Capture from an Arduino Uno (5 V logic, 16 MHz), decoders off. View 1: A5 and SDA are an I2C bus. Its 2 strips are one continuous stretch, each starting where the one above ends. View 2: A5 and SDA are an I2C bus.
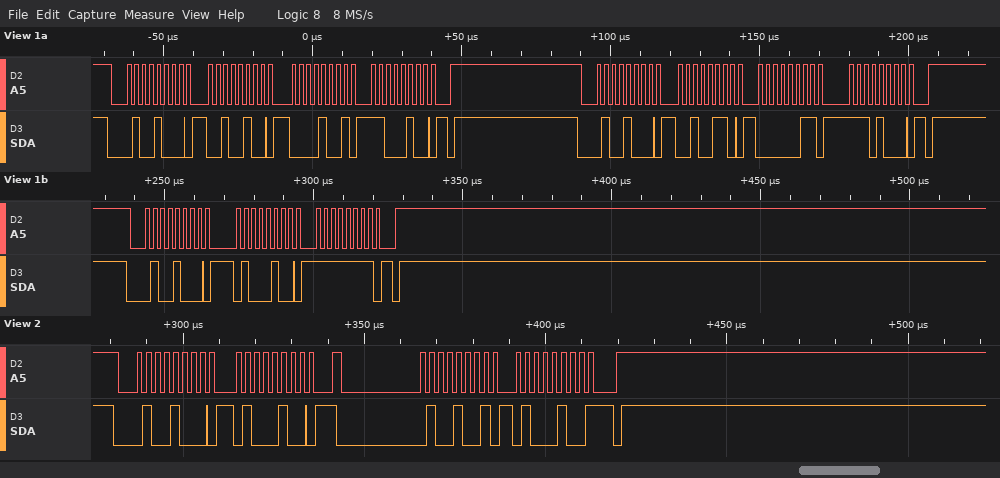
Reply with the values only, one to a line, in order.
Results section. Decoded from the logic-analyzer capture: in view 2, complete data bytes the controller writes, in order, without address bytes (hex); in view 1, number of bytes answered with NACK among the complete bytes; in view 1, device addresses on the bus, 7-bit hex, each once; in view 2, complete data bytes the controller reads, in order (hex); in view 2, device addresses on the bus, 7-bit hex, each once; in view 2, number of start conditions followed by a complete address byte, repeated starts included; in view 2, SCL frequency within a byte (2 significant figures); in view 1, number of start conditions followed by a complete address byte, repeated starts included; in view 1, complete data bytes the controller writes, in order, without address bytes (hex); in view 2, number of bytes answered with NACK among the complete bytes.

44
0
0x24
44
0x24
2
400 kHz
3
24 09 C4 26 03 E8 44 FF
1
